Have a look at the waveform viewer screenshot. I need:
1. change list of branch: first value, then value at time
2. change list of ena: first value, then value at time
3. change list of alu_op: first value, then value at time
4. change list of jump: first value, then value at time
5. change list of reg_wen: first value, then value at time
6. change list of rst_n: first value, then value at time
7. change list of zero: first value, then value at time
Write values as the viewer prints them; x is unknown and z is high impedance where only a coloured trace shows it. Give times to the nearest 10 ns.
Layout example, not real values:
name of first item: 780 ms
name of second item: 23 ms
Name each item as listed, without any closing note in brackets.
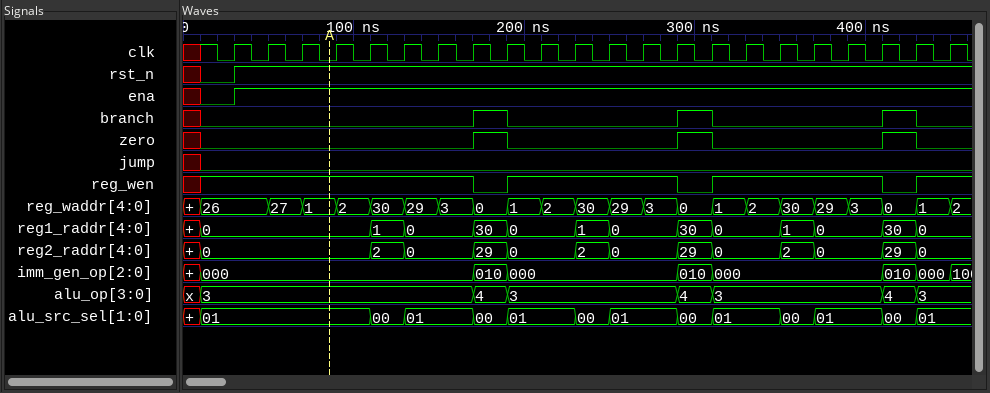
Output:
change list of branch: first value, then value at time: x, 0 at 10 ns, 1 at 170 ns, 0 at 190 ns, 1 at 290 ns, 0 at 310 ns, 1 at 410 ns, 0 at 430 ns
change list of ena: first value, then value at time: x, 0 at 10 ns, 1 at 30 ns
change list of alu_op: first value, then value at time: x, 3 at 10 ns, 4 at 170 ns, 3 at 190 ns, 4 at 290 ns, 3 at 310 ns, 4 at 410 ns, 3 at 430 ns
change list of jump: first value, then value at time: x, 0 at 10 ns
change list of reg_wen: first value, then value at time: x, 1 at 10 ns, 0 at 170 ns, 1 at 190 ns, 0 at 290 ns, 1 at 310 ns, 0 at 410 ns, 1 at 430 ns
change list of rst_n: first value, then value at time: x, 0 at 10 ns, 1 at 30 ns
change list of zero: first value, then value at time: x, 0 at 10 ns, 1 at 170 ns, 0 at 190 ns, 1 at 290 ns, 0 at 310 ns, 1 at 410 ns, 0 at 430 ns
